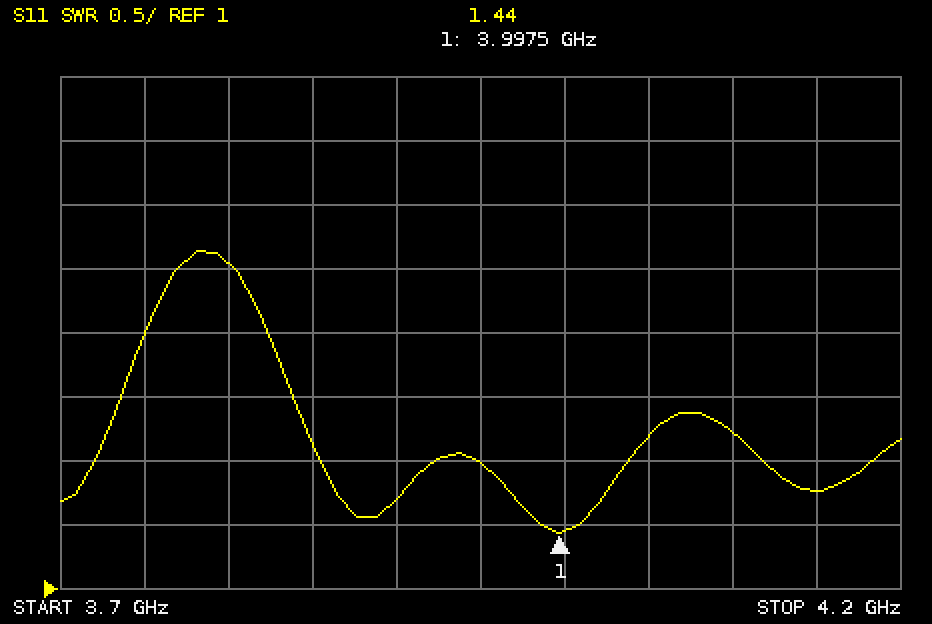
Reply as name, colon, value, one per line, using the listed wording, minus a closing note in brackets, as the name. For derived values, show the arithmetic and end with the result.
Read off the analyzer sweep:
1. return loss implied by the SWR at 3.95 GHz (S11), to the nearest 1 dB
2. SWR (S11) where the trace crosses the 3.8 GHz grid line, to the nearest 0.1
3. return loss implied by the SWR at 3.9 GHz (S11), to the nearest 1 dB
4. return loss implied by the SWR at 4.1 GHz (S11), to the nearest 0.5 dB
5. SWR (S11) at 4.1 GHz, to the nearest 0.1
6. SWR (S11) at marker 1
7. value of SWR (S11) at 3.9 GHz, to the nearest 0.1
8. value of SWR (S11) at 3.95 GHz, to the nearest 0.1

return loss implied by the SWR at 3.95 GHz (S11), to the nearest 1 dB: −20 log10((2 − 1)/(2 + 1)) ≈ 10 dB
SWR (S11) where the trace crosses the 3.8 GHz grid line, to the nearest 0.1: 3.5
return loss implied by the SWR at 3.9 GHz (S11), to the nearest 1 dB: −20 log10((1.7 − 1)/(1.7 + 1)) ≈ 12 dB
return loss implied by the SWR at 4.1 GHz (S11), to the nearest 0.5 dB: −20 log10((2.2 − 1)/(2.2 + 1)) ≈ 8.5 dB
SWR (S11) at 4.1 GHz, to the nearest 0.1: 2.2
SWR (S11) at marker 1: 1.44
value of SWR (S11) at 3.9 GHz, to the nearest 0.1: 1.7
value of SWR (S11) at 3.95 GHz, to the nearest 0.1: 2.0
